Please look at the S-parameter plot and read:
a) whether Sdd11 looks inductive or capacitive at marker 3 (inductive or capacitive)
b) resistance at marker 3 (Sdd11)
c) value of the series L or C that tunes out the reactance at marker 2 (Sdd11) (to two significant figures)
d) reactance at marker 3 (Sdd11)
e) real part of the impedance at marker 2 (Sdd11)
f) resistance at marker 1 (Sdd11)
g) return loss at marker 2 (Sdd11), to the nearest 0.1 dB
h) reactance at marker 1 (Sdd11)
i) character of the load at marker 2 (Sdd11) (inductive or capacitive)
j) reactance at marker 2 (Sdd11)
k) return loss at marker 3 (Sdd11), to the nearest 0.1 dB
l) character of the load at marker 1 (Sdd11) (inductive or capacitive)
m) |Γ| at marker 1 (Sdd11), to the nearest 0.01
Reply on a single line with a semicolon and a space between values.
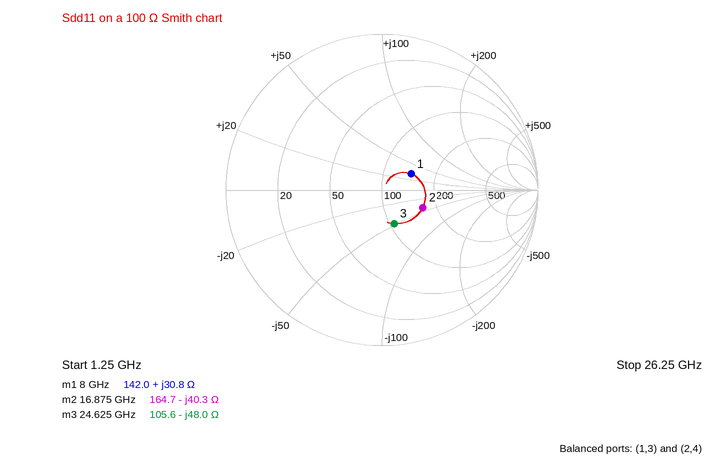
capacitive; 105.6 Ω; 380 pH; -48.0 Ω; 164.7 Ω; 142.0 Ω; 10.9 dB; +30.8 Ω; capacitive; -40.3 Ω; 12.8 dB; inductive; 0.21
